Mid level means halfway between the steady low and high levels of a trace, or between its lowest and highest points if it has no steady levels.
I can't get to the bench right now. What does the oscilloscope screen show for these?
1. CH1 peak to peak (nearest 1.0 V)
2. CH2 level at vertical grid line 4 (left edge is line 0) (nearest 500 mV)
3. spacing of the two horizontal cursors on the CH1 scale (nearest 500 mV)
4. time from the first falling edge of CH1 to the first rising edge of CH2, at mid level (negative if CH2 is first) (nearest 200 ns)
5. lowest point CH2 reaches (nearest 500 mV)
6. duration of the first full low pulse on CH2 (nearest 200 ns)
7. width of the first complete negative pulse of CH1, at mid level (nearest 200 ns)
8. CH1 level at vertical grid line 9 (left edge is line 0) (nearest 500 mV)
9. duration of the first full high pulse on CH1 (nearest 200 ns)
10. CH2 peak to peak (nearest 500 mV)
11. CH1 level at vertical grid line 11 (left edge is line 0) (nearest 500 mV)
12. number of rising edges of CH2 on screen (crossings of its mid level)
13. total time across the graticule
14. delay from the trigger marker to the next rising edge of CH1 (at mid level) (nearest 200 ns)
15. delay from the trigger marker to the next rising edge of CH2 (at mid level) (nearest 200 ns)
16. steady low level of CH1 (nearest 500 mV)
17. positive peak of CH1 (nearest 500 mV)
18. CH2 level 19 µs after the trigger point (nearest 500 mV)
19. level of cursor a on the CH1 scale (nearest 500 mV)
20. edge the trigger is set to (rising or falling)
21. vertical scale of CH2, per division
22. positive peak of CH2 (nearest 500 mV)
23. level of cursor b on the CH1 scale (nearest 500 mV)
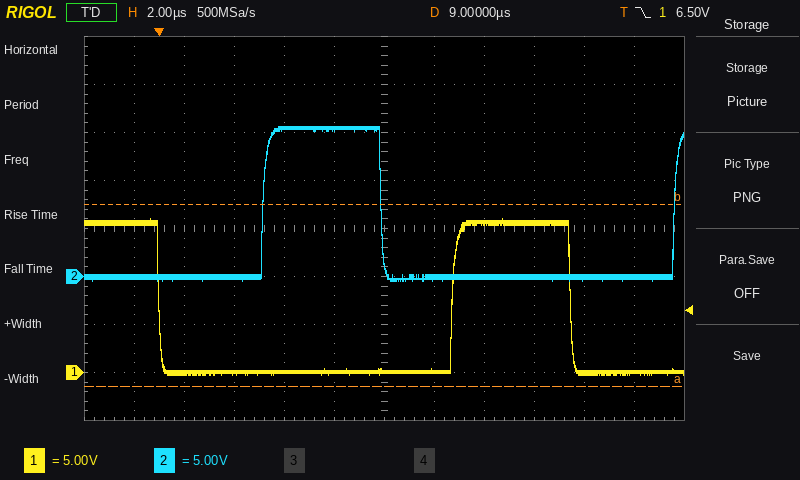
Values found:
16.0 V
15.5 V
19.0 V
+4.2 µs
-500 mV
11.8 µs
11.8 µs
15.5 V
4.8 µs
16.0 V
0.0 V
2
24 µs
11.8 µs
4.2 µs
0.0 V
16.0 V
0.0 V
-1.5 V
falling
5 V
15.5 V
17.5 V
